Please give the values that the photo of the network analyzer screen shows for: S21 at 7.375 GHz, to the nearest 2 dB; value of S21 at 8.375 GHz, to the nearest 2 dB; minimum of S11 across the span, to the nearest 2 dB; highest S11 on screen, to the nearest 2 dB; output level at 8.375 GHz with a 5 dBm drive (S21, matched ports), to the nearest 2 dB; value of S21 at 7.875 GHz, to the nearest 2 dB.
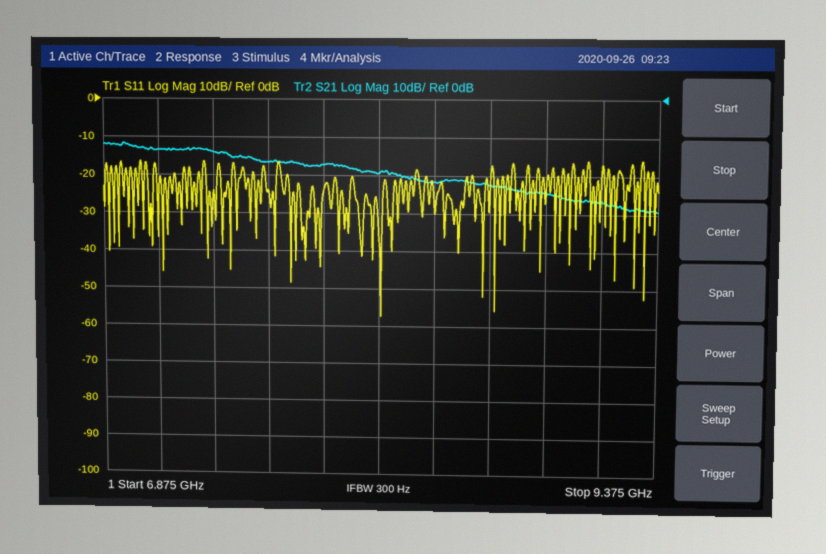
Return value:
-14 dB
-22 dB
-58 dB
-16 dB
-16 dBm
-18 dB
